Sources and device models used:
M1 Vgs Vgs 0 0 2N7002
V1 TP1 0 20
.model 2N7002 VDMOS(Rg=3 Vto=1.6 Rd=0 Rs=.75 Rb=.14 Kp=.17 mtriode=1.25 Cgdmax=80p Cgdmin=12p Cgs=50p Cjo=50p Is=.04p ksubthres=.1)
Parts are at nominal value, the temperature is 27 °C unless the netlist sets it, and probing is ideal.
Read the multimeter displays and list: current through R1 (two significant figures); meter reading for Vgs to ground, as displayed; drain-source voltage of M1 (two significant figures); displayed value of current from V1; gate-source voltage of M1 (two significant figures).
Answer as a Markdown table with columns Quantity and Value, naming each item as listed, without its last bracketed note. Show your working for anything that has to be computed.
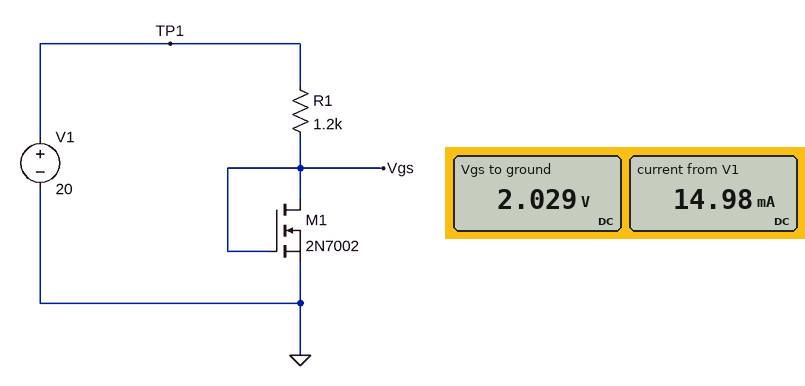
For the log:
| Quantity | Value |
|---|---|
| current through R1 | (20 V - 2.029 V) / 1.2 kΩ = 15 mA |
| meter reading for Vgs to ground, as displayed | 2.029 V |
| drain-source voltage of M1 | 2.029 V = 2.0 V |
| displayed value of current from V1 | 14.98 mA |
| gate-source voltage of M1 | 2.029 V = 2.0 V |
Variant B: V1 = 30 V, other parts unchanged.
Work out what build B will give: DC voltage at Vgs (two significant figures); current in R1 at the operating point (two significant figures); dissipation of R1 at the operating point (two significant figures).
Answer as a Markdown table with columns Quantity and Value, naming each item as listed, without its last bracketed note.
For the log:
| Quantity | Value |
|---|---|
| DC voltage at Vgs | 2.1 V |
| current in R1 at the operating point | 23 mA |
| dissipation of R1 at the operating point | 650 mW |
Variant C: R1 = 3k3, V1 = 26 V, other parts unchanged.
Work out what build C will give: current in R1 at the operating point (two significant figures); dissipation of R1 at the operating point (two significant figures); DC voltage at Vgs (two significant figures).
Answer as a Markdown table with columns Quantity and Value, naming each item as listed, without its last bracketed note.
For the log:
| Quantity | Value |
|---|---|
| current in R1 at the operating point | 7.3 mA |
| dissipation of R1 at the operating point | 180 mW |
| DC voltage at Vgs | 1.9 V |
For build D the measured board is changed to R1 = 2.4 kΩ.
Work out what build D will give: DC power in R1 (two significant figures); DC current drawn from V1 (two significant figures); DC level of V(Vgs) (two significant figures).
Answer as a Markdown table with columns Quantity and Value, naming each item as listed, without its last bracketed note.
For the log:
| Quantity | Value |
|---|---|
| DC power in R1 | 140 mW |
| DC current drawn from V1 | 7.5 mA |
| DC level of V(Vgs) | 1.9 V |
